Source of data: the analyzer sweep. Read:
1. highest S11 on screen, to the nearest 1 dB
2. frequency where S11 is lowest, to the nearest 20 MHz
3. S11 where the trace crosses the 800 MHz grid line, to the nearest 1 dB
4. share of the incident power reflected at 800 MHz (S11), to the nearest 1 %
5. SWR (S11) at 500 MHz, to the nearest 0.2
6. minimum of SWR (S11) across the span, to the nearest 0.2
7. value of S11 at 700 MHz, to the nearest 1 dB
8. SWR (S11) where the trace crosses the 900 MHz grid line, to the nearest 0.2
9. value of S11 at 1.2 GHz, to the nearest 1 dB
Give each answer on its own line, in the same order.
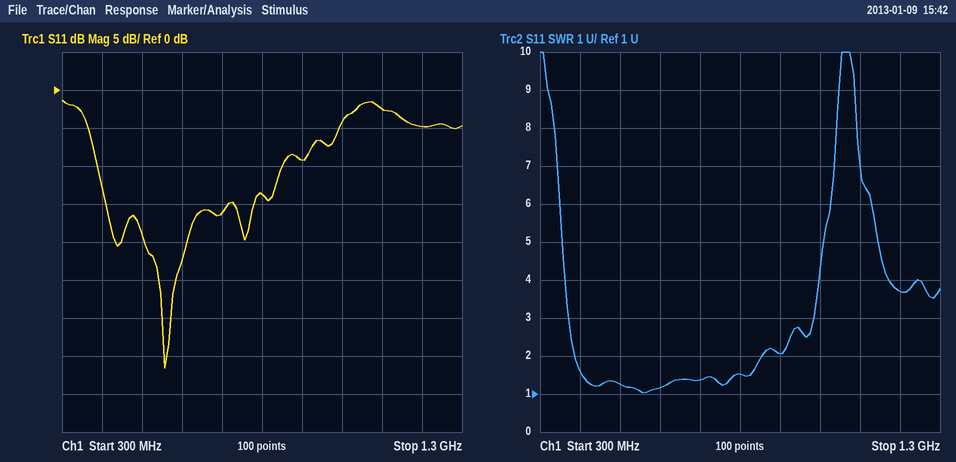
-1 dB
560 MHz
-14 dB
4 %
1.2
1.0
-16 dB
2.0
-5 dB
